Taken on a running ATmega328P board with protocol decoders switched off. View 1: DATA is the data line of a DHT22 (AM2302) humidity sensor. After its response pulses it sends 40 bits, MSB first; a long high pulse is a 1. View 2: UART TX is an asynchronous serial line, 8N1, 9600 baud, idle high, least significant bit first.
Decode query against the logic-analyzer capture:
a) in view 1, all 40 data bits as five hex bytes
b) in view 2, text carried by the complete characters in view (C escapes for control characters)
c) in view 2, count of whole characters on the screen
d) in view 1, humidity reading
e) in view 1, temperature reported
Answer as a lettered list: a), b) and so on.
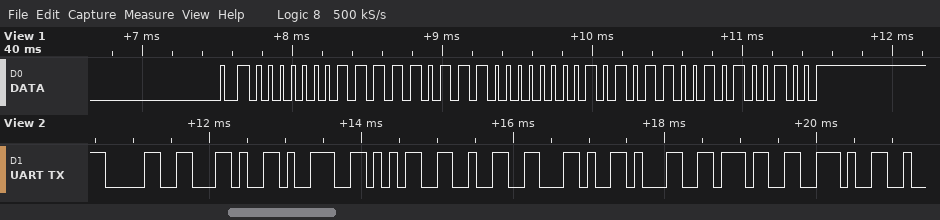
a) 01 F7 00 AC A4
b) "0,952,17."
c) 9
d) 50.3 %
e) 17.2 °C
